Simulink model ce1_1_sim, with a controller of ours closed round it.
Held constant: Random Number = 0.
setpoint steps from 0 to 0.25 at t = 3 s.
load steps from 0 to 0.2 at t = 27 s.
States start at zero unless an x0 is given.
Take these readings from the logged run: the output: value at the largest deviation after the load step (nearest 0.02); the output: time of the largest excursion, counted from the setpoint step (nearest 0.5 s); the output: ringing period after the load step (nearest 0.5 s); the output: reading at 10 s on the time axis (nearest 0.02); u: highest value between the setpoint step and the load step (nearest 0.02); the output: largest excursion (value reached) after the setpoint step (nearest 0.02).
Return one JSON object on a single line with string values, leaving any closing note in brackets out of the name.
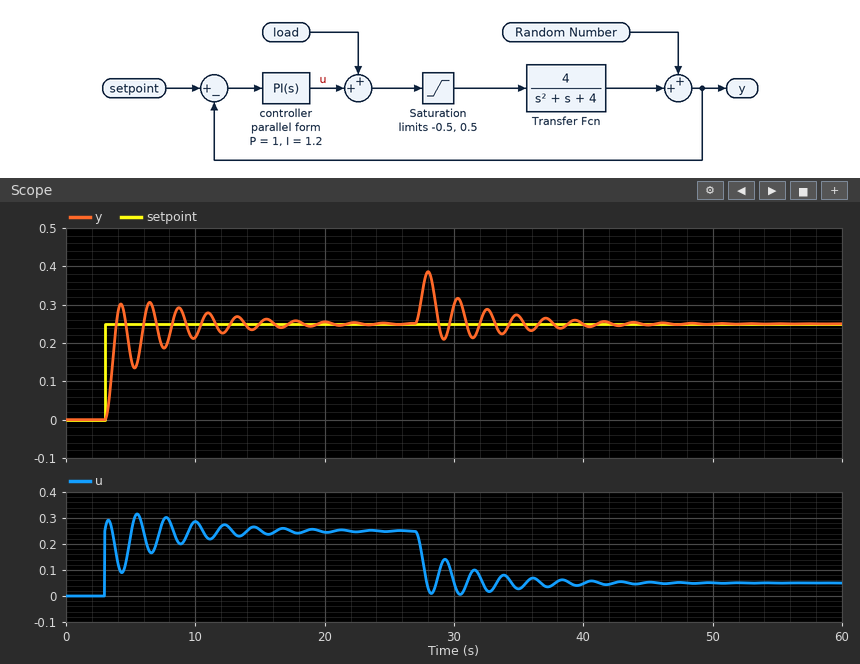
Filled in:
{"the output: value at the largest deviation after the load step": "0.38", "the output: time of the largest excursion, counted from the setpoint step": "3.5 s", "the output: ringing period after the load step": "2.5 s", "the output: reading at 10 s on the time axis": "0.22", "u: highest value between the setpoint step and the load step": "0.32", "the output: largest excursion (value reached) after the setpoint step": "0.30"}
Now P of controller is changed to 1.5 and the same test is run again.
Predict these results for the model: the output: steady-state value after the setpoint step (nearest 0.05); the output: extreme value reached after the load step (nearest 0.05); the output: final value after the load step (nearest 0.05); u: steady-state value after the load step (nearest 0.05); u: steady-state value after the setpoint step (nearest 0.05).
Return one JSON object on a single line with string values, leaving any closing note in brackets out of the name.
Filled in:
{"the output: steady-state value after the setpoint step": "0.25", "the output: extreme value reached after the load step": "0.35", "the output: final value after the load step": "0.25", "u: steady-state value after the load step": "0.05", "u: steady-state value after the setpoint step": "0.25"}
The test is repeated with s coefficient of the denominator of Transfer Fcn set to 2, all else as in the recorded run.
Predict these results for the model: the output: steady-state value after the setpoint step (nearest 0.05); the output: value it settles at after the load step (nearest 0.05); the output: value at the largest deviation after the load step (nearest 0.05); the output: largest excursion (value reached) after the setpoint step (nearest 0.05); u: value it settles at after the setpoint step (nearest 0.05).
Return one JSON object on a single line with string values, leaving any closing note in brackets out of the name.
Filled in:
{"the output: steady-state value after the setpoint step": "0.25", "the output: value it settles at after the load step": "0.25", "the output: value at the largest deviation after the load step": "0.35", "the output: largest excursion (value reached) after the setpoint step": "0.25", "u: value it settles at after the setpoint step": "0.25"}
